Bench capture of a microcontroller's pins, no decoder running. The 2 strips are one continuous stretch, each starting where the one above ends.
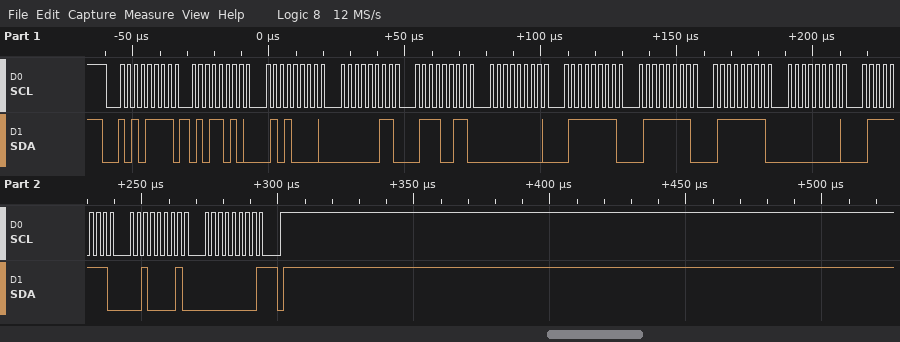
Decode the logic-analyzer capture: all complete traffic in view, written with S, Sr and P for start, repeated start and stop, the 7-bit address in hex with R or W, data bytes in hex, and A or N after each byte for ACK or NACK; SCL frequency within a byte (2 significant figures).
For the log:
S 57R A 5A A 50 A 03 A 73 A 00 A 7F A 7F A 7F A 00 A 7F A 21 A 00 N P
400 kHz
